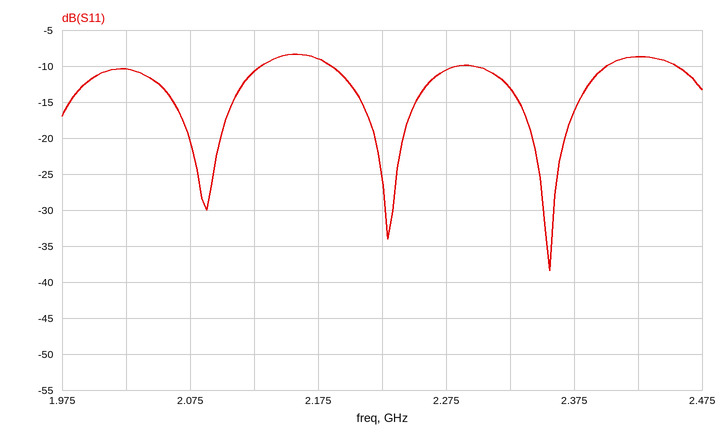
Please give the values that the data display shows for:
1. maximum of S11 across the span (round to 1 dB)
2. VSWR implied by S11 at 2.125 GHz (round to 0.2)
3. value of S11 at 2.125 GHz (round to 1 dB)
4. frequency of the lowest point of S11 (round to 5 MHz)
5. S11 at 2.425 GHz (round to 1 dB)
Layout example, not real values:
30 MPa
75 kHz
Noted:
-8 dB
1.8
-11 dB
2.355 GHz
-9 dB
